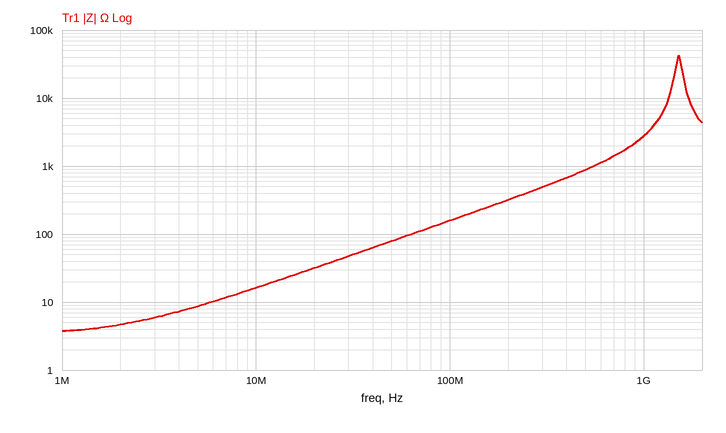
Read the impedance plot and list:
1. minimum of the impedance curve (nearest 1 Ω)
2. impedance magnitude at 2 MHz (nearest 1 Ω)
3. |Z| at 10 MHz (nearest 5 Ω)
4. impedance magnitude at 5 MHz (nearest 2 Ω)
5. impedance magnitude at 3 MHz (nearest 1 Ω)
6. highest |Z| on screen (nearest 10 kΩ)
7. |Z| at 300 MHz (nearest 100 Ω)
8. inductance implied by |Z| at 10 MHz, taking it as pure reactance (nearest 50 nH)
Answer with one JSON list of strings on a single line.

["4 Ω", "5 Ω", "15 Ω", "8 Ω", "6 Ω", "40 kΩ", "500 Ω", "250 nH"]
